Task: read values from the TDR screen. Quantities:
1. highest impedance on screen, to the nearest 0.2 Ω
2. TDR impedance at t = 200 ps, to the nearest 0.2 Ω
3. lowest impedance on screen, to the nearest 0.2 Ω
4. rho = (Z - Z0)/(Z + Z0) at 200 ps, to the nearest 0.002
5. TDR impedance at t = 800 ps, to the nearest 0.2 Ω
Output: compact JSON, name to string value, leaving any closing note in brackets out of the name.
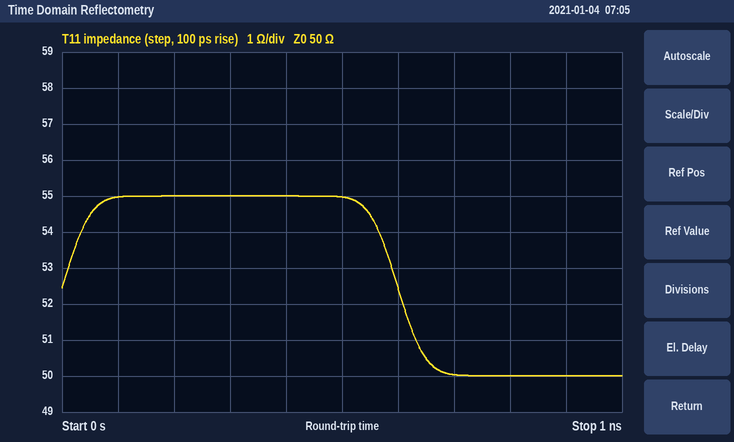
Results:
{"highest impedance on screen, to the nearest 0.2 Ω": "55.0 Ω", "TDR impedance at t = 200 ps, to the nearest 0.2 Ω": "55.0 Ω", "lowest impedance on screen, to the nearest 0.2 Ω": "50.0 Ω", "rho = (Z - Z0)/(Z + Z0) at 200 ps, to the nearest 0.002": "+0.048", "TDR impedance at t = 800 ps, to the nearest 0.2 Ω": "50.0 Ω"}
